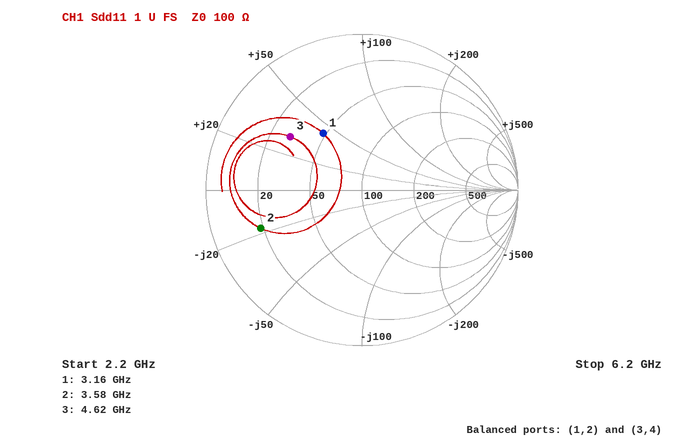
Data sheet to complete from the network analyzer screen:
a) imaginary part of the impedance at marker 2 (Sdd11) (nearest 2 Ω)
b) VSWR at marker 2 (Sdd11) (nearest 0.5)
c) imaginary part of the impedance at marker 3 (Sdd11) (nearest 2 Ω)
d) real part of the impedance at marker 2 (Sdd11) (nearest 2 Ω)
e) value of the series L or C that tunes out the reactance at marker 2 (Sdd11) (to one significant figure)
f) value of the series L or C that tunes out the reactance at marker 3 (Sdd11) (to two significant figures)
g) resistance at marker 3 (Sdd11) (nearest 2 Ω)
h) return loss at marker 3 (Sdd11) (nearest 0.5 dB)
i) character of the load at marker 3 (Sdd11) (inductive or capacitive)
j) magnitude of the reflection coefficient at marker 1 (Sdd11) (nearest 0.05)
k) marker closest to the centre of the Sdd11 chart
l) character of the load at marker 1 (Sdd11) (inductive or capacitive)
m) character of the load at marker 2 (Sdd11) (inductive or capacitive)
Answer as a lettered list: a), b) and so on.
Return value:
a) -18 Ω
b) 5.5
c) +30 Ω
d) 18 Ω
e) 800 pH
f) 1.1 pF
g) 30 Ω
h) 5.0 dB
i) inductive
j) 0.45
k) marker 1
l) inductive
m) capacitive
